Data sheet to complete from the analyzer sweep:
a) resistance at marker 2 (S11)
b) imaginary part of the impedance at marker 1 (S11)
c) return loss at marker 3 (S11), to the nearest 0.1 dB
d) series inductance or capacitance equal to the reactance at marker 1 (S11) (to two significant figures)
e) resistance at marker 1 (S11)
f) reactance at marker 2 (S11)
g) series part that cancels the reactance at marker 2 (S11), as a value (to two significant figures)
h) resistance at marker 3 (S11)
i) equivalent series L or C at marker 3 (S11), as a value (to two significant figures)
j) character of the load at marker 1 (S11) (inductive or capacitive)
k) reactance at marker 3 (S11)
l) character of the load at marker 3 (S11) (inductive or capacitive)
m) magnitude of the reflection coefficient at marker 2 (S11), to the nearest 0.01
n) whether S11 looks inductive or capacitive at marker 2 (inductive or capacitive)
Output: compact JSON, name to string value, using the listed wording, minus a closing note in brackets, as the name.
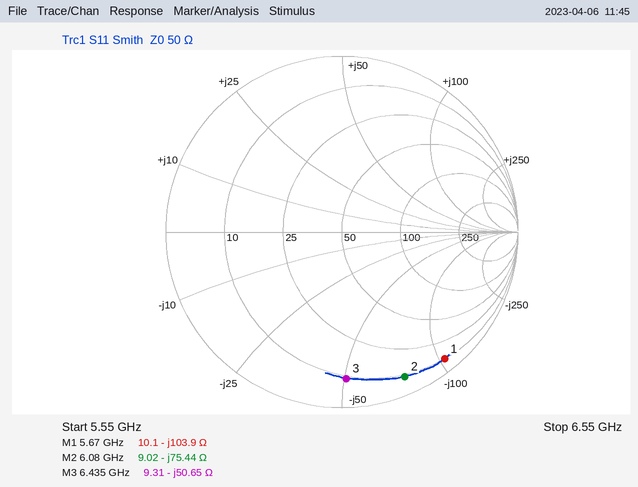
{"resistance at marker 2": "9.02 Ω", "imaginary part of the impedance at marker 1": "-103.9 Ω", "return loss at marker 3 (S11), to the nearest 0.1 dB": "1.6 dB", "series inductance or capacitance equal to the reactance at marker 1 (S11)": "270 fF", "resistance at marker 1": "10.1 Ω", "reactance at marker 2": "-75.44 Ω", "series part that cancels the reactance at marker 2 (S11), as a value": "2.0 nH", "resistance at marker 3": "9.31 Ω", "equivalent series L or C at marker 3 (S11), as a value": "490 fF", "character of the load at marker 1 (S11)": "capacitive", "reactance at marker 3": "-50.65 Ω", "character of the load at marker 3 (S11)": "capacitive", "magnitude of the reflection coefficient at marker 2 (S11), to the nearest 0.01": "0.90", "whether S11 looks inductive or capacitive at marker 2": "capacitive"}
